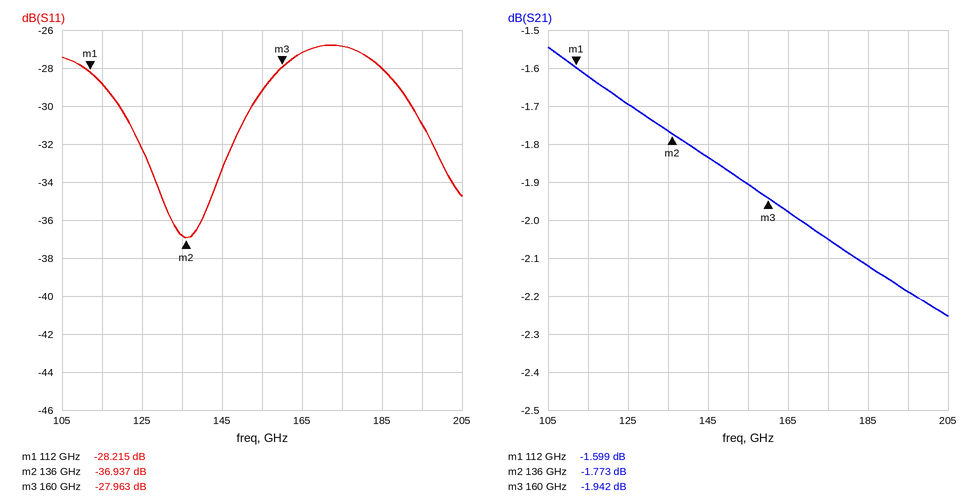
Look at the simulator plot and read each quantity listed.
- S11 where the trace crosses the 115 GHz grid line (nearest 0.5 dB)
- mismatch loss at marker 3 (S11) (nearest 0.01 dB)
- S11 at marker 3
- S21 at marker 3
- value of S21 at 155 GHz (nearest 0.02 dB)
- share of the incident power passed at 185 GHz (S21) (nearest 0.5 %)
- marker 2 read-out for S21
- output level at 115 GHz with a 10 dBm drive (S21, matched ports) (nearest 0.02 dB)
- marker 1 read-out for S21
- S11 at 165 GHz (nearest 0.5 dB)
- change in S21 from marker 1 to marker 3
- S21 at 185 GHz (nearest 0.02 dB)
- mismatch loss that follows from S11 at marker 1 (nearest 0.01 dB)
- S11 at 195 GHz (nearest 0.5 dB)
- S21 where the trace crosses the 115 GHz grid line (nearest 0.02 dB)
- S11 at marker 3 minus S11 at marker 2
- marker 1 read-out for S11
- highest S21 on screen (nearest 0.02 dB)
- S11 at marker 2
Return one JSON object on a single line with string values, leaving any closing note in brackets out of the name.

{"S11 where the trace crosses the 115 GHz grid line": "-29.0 dB", "mismatch loss at marker 3 (S11)": "0.01 dB", "S11 at marker 3": "-27.963 dB", "S21 at marker 3": "-1.942 dB", "value of S21 at 155 GHz": "-1.90 dB", "share of the incident power passed at 185 GHz (S21)": "61.5 %", "marker 2 read-out for S21": "-1.773 dB", "output level at 115 GHz with a 10 dBm drive (S21, matched ports)": "8.38 dBm", "marker 1 read-out for S21": "-1.599 dB", "S11 at 165 GHz": "-27.0 dB", "change in S21 from marker 1 to marker 3": "-0.343 dB", "S21 at 185 GHz": "-2.12 dB", "mismatch loss that follows from S11 at marker 1": "0.01 dB", "S11 at 195 GHz": "-31.0 dB", "S21 where the trace crosses the 115 GHz grid line": "-1.62 dB", "S11 at marker 3 minus S11 at marker 2": "8.974 dB", "marker 1 read-out for S11": "-28.215 dB", "highest S21 on screen": "-1.54 dB", "S11 at marker 2": "-36.937 dB"}
